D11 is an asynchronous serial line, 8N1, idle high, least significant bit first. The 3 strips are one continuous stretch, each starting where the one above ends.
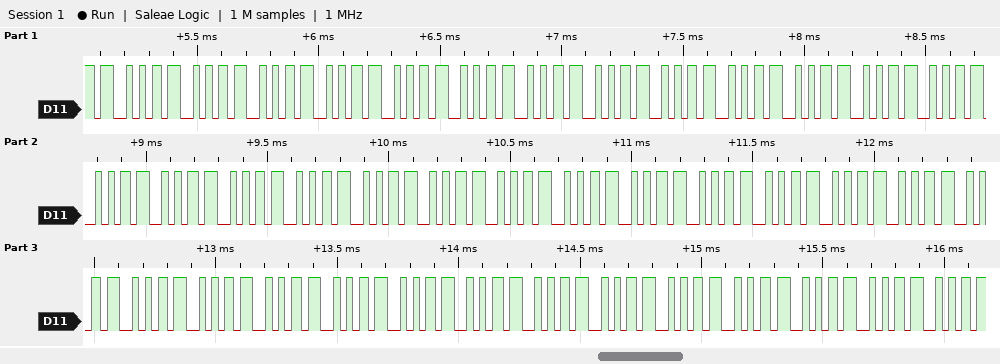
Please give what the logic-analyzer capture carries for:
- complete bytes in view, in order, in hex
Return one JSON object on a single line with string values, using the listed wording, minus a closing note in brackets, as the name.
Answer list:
{"complete bytes in view, in order, in hex": "53 53 53 53 53 53 53 53 53 53 53 53 53 53 53 53 53 53 53 53 53 53 53 53 53 53 53 53 53 53 53 53 53 53 53 53 53 53 53 53"}
